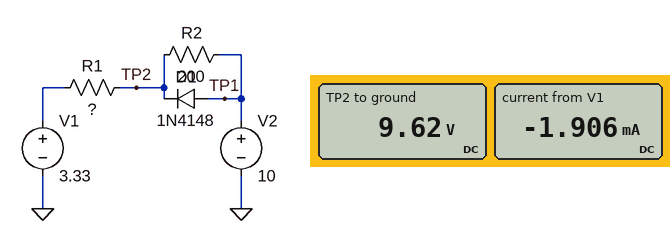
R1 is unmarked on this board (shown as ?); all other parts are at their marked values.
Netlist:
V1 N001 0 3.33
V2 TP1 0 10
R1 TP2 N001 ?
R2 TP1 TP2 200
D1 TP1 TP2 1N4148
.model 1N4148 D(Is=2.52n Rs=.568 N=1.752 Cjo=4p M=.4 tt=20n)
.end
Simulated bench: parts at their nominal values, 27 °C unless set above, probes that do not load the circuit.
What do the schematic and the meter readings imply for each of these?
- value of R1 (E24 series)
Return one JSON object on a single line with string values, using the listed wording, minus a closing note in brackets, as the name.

{"value of R1": "3.3 kΩ"}
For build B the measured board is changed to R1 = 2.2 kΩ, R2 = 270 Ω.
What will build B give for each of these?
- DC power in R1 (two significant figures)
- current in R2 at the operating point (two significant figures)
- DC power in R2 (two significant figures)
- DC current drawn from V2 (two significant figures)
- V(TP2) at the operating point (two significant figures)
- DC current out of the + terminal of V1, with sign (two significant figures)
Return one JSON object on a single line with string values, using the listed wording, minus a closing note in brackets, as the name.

{"DC power in R1": "17 mW", "current in R2 at the operating point": "2.1 mA", "DC power in R2": "1.2 mW", "DC current drawn from V2": "2.8 mA", "V(TP2) at the operating point": "9.4 V", "DC current out of the + terminal of V1, with sign": "-2.8 mA"}
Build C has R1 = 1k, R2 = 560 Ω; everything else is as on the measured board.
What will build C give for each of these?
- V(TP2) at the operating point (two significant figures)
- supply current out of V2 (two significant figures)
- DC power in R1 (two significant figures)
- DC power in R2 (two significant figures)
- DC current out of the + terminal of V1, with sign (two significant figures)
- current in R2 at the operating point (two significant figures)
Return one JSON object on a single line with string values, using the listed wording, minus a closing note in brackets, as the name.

{"V(TP2) at the operating point": "9.3 V", "supply current out of V2": "6.0 mA", "DC power in R1": "36 mW", "DC power in R2": "770 µW", "DC current out of the + terminal of V1, with sign": "-6.0 mA", "current in R2 at the operating point": "1.2 mA"}
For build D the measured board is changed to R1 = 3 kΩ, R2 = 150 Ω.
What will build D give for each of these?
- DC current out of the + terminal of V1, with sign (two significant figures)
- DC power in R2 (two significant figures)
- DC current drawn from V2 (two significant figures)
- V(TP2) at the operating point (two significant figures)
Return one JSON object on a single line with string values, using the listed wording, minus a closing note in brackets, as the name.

{"DC current out of the + terminal of V1, with sign": "-2.1 mA", "DC power in R2": "670 µW", "DC current drawn from V2": "2.1 mA", "V(TP2) at the operating point": "9.7 V"}
